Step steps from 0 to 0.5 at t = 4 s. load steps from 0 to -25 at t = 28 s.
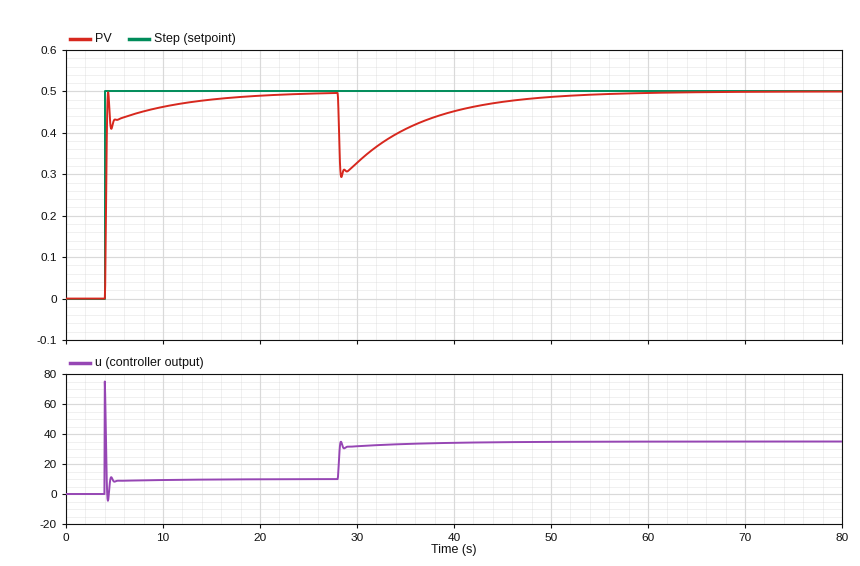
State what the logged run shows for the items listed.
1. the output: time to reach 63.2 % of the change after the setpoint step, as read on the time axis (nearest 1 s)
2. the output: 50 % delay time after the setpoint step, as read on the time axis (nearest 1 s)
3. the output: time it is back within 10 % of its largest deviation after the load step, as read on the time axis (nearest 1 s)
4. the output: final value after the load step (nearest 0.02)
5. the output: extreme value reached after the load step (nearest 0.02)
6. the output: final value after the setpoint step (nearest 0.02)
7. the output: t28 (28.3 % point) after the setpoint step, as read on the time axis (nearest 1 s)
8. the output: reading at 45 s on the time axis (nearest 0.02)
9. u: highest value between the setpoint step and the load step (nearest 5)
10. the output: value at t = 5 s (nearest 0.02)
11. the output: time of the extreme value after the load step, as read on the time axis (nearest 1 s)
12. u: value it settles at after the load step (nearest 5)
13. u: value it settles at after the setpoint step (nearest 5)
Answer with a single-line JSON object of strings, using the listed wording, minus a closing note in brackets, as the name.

{"the output: time to reach 63.2 % of the change after the setpoint step, as read on the time axis": "4 s", "the output: 50 % delay time after the setpoint step, as read on the time axis": "4 s", "the output: time it is back within 10 % of its largest deviation after the load step, as read on the time axis": "47 s", "the output: final value after the load step": "0.50", "the output: extreme value reached after the load step": "0.30", "the output: final value after the setpoint step": "0.50", "the output: t28 (28.3 % point) after the setpoint step, as read on the time axis": "4 s", "the output: reading at 45 s on the time axis": "0.48", "u: highest value between the setpoint step and the load step": "75", "the output: value at t = 5 s": "0.44", "the output: time of the extreme value after the load step, as read on the time axis": "28 s", "u: value it settles at after the load step": "35", "u: value it settles at after the setpoint step": "10"}
